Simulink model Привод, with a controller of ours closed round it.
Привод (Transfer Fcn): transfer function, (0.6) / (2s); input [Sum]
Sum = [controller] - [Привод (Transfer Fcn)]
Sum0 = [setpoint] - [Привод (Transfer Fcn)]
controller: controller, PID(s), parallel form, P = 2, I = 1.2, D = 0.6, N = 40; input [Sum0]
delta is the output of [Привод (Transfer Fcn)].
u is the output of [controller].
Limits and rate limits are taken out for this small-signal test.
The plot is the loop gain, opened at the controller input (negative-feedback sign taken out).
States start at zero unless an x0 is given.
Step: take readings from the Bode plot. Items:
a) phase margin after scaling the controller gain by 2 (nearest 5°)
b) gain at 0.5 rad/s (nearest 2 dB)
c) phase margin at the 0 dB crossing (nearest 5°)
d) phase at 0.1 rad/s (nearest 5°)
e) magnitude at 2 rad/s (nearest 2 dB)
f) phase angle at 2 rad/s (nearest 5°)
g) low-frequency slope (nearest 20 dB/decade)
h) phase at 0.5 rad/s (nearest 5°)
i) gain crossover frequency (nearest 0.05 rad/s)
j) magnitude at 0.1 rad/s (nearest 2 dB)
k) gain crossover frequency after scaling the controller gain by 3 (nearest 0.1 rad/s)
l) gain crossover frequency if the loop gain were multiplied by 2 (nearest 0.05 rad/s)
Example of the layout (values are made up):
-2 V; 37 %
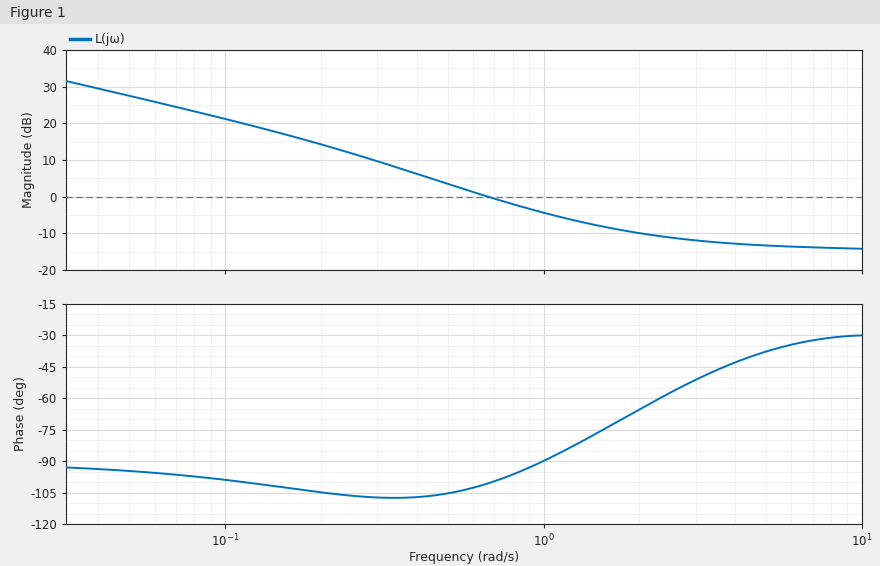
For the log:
95°; 4 dB; 80°; -100°; -10 dB; -65°; -20 dB/decade; -105°; 0.65 rad/s; 22 dB; 1.9 rad/s; 1.20 rad/s
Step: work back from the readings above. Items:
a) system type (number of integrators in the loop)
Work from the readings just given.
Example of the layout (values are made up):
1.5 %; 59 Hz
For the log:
1
